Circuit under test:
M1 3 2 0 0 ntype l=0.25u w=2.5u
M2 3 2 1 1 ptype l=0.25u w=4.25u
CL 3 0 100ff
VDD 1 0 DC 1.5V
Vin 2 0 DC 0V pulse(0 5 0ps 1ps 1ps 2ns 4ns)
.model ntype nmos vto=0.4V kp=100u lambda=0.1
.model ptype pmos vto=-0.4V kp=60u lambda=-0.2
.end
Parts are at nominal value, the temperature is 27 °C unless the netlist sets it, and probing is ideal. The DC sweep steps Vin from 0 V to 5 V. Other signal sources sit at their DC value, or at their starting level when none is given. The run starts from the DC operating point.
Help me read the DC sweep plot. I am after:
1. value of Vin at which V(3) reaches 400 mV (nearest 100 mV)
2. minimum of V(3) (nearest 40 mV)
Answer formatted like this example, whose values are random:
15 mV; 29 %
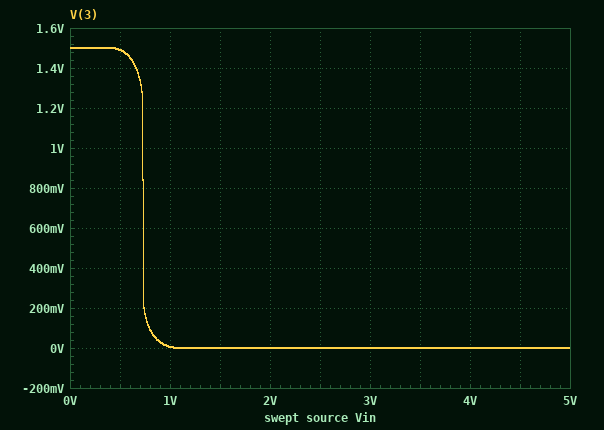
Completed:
700 mV; 0 V
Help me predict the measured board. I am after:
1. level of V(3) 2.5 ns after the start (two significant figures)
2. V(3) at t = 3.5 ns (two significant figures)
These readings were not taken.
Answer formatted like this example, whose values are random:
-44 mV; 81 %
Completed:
1.5 V; 1.5 V
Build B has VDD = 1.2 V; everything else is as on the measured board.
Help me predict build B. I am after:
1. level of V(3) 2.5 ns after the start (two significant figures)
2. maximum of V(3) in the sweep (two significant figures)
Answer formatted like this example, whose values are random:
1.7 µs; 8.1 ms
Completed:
1.1 V; 1.2 V
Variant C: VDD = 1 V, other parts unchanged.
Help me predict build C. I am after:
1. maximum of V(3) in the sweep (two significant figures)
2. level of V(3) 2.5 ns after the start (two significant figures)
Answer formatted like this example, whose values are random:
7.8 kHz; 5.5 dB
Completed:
1.0 V; 750 mV
